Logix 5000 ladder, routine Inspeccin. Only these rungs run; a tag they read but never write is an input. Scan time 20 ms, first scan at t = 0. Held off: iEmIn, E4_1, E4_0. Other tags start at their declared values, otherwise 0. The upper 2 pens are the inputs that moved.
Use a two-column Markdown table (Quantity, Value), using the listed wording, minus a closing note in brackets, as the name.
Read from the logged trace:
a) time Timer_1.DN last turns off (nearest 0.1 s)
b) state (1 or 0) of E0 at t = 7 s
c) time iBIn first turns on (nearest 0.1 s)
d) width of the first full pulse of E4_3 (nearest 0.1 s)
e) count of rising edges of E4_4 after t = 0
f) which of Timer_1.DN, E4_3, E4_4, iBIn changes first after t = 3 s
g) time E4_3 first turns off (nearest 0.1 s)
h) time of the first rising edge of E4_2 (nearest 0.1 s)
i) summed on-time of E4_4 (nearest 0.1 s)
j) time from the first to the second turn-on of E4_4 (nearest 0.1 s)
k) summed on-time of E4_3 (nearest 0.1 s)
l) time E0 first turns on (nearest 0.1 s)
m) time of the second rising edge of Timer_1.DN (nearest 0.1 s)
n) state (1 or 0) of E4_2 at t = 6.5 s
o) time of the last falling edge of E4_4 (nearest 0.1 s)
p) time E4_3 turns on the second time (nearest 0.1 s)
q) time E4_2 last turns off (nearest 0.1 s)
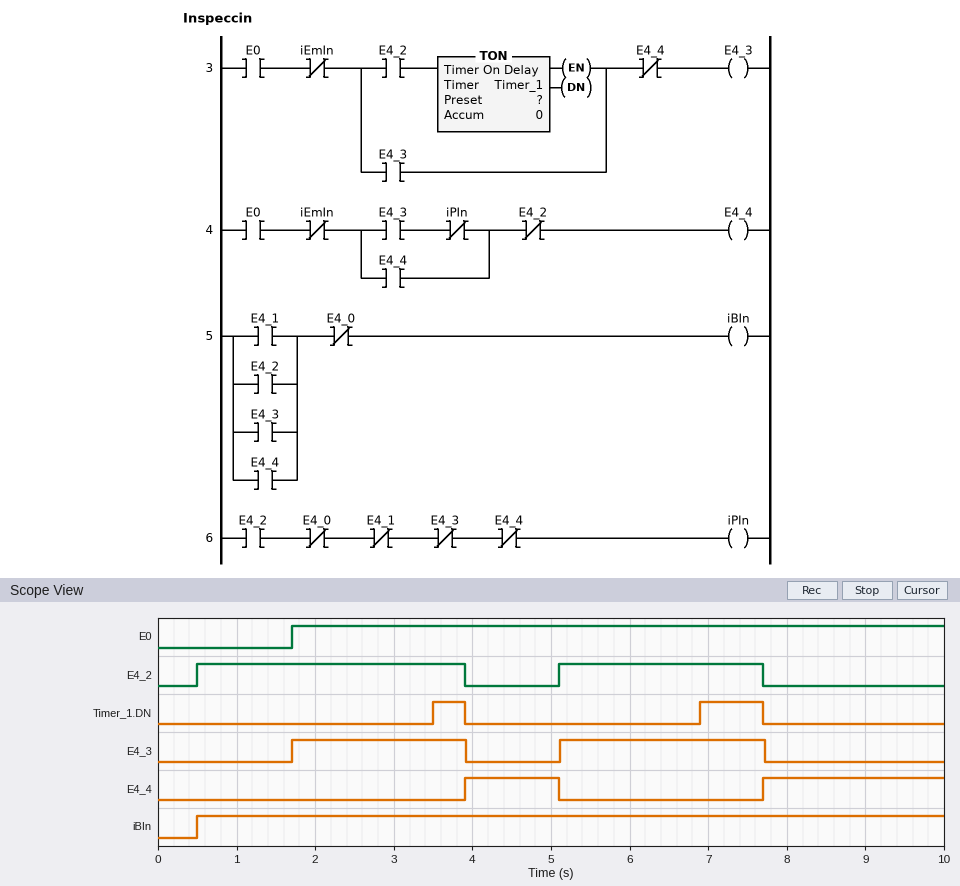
| Quantity | Value |
|---|---|
| time Timer_1.DN last turns off | 7.7 s |
| state (1 or 0) of E0 at t = 7 s | 1 |
| time iBIn first turns on | 0.5 s |
| width of the first full pulse of E4_3 | 2.2 s |
| count of rising edges of E4_4 after t = 0 | 2 |
| which of Timer_1.DN, E4_3, E4_4, iBIn changes first after t = 3 s | Timer_1.DN |
| time E4_3 first turns off | 3.9 s |
| time of the first rising edge of E4_2 | 0.5 s |
| summed on-time of E4_4 | 3.5 s |
| time from the first to the second turn-on of E4_4 | 3.8 s |
| summed on-time of E4_3 | 4.8 s |
| time E0 first turns on | 1.7 s |
| time of the second rising edge of Timer_1.DN | 6.9 s |
| state (1 or 0) of E4_2 at t = 6.5 s | 1 |
| time of the last falling edge of E4_4 | 5.1 s |
| time E4_3 turns on the second time | 5.1 s |
| time E4_2 last turns off | 7.7 s |
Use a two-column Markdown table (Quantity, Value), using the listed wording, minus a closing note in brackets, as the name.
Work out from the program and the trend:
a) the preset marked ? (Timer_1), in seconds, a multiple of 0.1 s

| Quantity | Value |
|---|---|
| the preset marked ? (Timer_1), in seconds, a multiple of 0.1 s | 1.8 s |
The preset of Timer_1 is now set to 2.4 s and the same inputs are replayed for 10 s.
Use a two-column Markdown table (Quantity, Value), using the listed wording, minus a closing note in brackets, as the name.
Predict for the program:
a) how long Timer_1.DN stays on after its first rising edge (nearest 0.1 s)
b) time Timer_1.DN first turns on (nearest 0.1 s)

| Quantity | Value |
|---|---|
| how long Timer_1.DN stays on after its first rising edge | 0.2 s |
| time Timer_1.DN first turns on | 7.5 s |
